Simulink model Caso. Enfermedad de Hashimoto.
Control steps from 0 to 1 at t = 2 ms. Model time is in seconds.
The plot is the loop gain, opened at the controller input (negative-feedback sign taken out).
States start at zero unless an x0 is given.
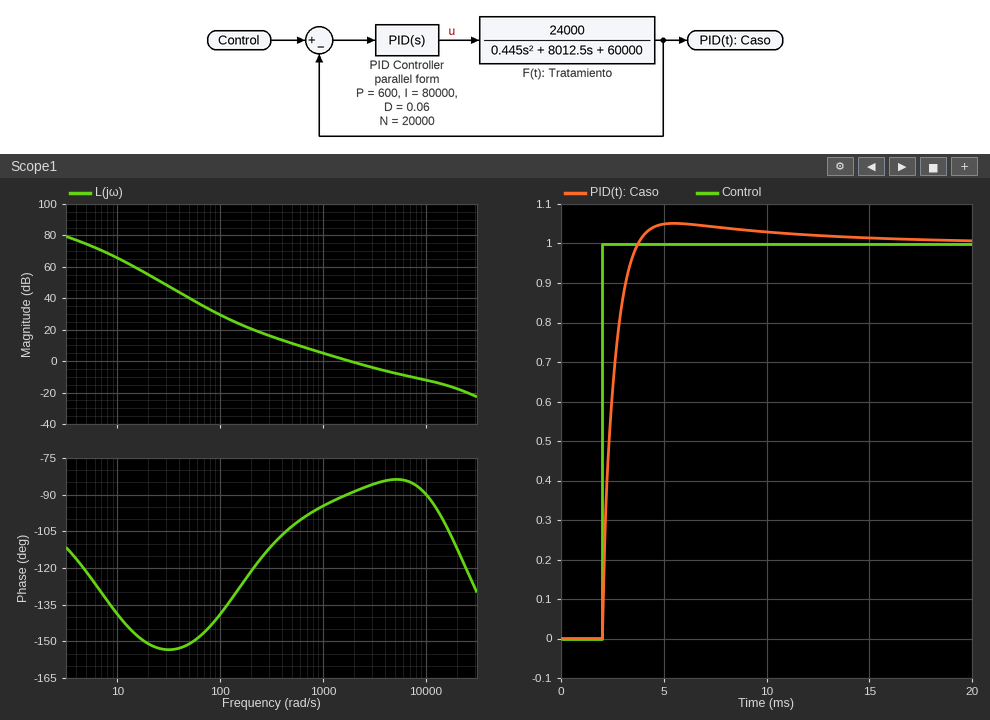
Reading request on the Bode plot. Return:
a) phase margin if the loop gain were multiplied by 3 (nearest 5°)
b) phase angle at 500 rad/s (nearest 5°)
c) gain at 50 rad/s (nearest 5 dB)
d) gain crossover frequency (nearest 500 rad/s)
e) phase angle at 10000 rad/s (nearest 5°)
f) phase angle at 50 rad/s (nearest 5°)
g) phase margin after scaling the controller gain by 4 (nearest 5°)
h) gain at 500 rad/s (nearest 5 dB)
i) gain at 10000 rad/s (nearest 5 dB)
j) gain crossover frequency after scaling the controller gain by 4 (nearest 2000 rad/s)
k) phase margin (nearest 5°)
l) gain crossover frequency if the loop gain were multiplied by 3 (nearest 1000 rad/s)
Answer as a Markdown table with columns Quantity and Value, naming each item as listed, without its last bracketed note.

| Quantity | Value |
|---|---|
| phase margin if the loop gain were multiplied by 3 | 95° |
| phase angle at 500 rad/s | -105° |
| gain at 50 rad/s | 40 dB |
| gain crossover frequency | 2000 rad/s |
| phase angle at 10000 rad/s | -90° |
| phase angle at 50 rad/s | -150° |
| phase margin after scaling the controller gain by 4 | 90° |
| gain at 500 rad/s | 10 dB |
| gain at 10000 rad/s | -10 dB |
| gain crossover frequency after scaling the controller gain by 4 | 10000 rad/s |
| phase margin | 90° |
| gain crossover frequency if the loop gain were multiplied by 3 | 7000 rad/s |
